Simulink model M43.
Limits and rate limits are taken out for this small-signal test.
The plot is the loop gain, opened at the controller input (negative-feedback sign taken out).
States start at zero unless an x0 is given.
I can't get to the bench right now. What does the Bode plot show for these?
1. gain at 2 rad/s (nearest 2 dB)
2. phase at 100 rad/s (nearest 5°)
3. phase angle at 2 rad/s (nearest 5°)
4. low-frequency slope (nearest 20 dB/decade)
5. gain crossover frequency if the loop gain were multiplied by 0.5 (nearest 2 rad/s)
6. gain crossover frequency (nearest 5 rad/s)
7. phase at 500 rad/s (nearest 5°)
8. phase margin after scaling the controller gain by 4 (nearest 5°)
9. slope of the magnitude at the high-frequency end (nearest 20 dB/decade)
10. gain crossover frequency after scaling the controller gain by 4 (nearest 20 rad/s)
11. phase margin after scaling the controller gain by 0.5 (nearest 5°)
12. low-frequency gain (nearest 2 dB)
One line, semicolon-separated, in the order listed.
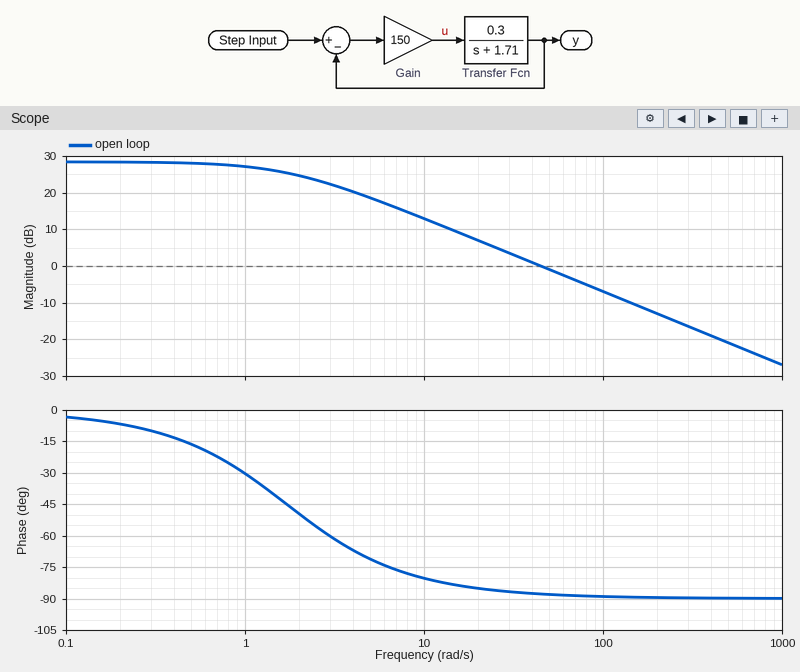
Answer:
24 dB; -90°; -50°; 0 dB/decade; 22 rad/s; 45 rad/s; -90°; 90°; -20 dB/decade; 180 rad/s; 95°; 28 dB
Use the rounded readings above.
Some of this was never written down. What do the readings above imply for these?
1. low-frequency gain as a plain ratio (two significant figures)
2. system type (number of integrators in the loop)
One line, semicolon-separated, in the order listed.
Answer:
25; 0
